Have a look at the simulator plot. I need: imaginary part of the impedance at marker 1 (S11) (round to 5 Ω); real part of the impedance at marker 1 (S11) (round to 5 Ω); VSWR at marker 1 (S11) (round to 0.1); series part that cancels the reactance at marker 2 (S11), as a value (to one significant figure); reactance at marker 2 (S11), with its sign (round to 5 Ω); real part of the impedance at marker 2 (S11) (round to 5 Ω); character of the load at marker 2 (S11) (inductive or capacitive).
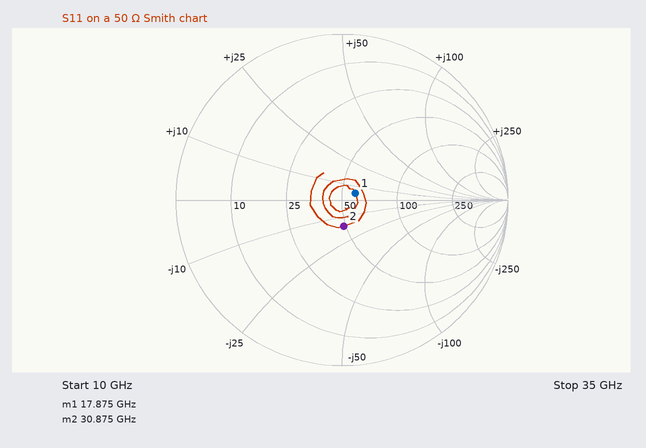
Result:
+5 Ω
60 Ω
1.2
80 pH
-15 Ω
50 Ω
capacitive
